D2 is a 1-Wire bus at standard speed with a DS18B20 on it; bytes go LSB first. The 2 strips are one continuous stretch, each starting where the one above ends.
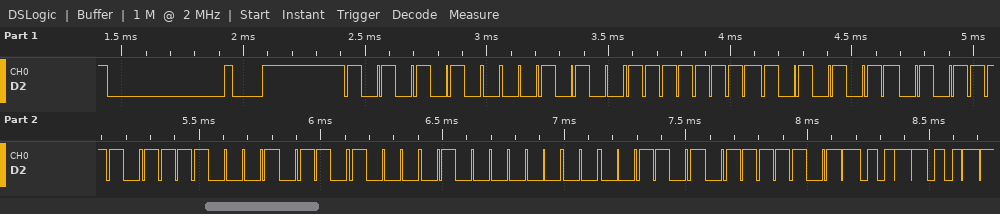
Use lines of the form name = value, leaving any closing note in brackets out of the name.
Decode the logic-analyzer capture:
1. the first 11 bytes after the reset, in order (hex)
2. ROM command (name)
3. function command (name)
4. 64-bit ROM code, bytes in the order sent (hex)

the first 11 bytes after the reset, in order = 55 28 FF D5 7A 8F 16 02 B0 BE 99
ROM command = Match ROM
function command = Read Scratchpad
64-bit ROM code, bytes in the order sent = 28 FF D5 7A 8F 16 02 B0
